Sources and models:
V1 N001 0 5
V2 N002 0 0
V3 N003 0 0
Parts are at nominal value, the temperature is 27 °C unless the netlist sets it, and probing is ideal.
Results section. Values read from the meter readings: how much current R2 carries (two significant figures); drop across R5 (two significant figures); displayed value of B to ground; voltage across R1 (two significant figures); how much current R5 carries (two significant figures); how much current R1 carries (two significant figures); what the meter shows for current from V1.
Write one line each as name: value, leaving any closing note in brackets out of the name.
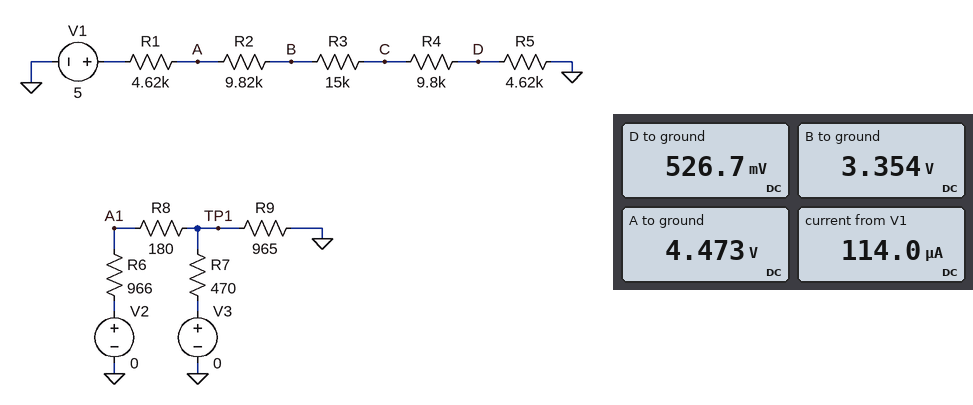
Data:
how much current R2 carries: 110 µA
drop across R5: 530 mV
displayed value of B to ground: 3.354 V
voltage across R1: 530 mV
how much current R5 carries: 110 µA
how much current R1 carries: 110 µA
what the meter shows for current from V1: 114.0 µA
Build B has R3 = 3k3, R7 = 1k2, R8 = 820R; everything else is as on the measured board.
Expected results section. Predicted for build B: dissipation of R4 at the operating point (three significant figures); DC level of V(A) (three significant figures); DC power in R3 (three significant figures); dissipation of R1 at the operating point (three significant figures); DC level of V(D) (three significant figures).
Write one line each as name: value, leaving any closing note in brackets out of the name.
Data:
dissipation of R4 at the operating point: 237 µW
DC level of V(A): 4.28 V
DC power in R3: 79.8 µW
dissipation of R1 at the operating point: 112 µW
DC level of V(D): 718 mV
